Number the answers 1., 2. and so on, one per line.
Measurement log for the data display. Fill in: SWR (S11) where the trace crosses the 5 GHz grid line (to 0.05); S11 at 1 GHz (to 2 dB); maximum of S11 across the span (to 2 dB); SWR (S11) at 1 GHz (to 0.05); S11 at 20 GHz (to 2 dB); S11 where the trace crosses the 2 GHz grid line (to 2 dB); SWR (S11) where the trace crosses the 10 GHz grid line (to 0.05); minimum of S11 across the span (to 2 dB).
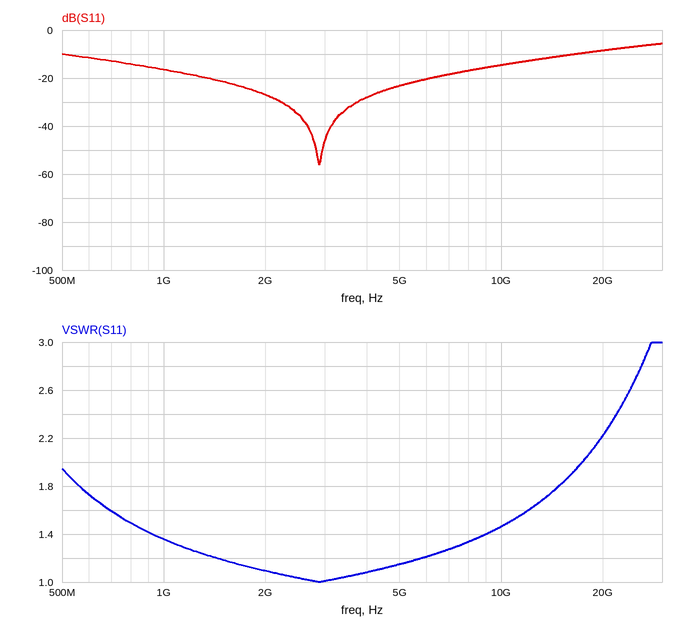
1. 1.15
2. -16 dB
3. -6 dB
4. 1.35
5. -8 dB
6. -26 dB
7. 1.45
8. -56 dB
